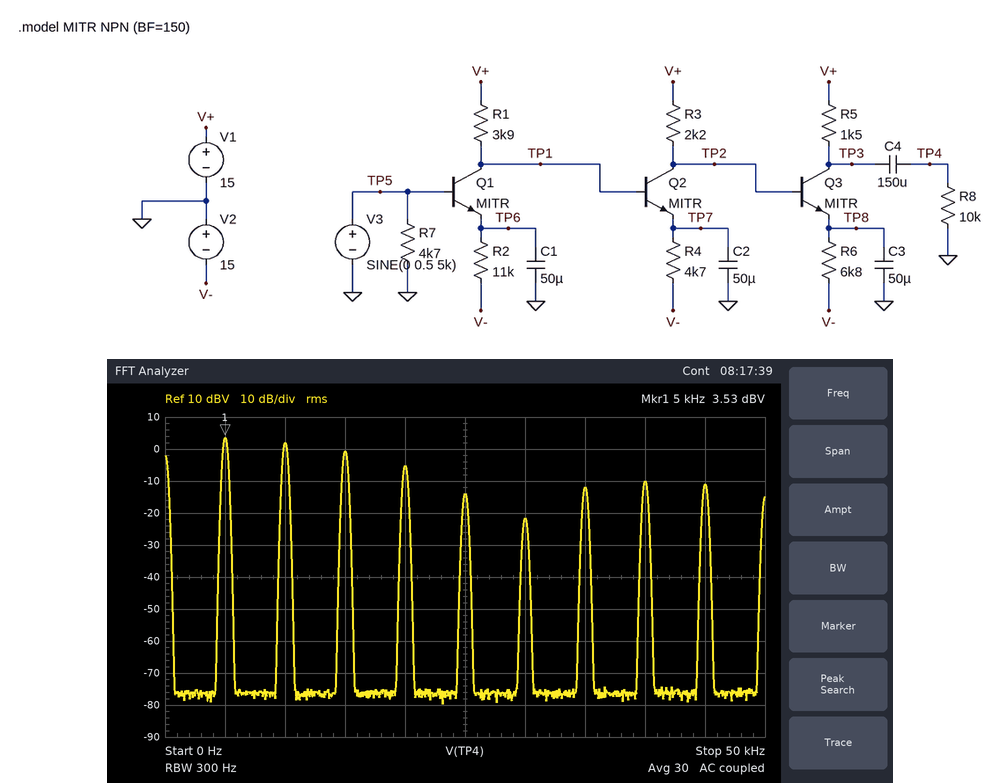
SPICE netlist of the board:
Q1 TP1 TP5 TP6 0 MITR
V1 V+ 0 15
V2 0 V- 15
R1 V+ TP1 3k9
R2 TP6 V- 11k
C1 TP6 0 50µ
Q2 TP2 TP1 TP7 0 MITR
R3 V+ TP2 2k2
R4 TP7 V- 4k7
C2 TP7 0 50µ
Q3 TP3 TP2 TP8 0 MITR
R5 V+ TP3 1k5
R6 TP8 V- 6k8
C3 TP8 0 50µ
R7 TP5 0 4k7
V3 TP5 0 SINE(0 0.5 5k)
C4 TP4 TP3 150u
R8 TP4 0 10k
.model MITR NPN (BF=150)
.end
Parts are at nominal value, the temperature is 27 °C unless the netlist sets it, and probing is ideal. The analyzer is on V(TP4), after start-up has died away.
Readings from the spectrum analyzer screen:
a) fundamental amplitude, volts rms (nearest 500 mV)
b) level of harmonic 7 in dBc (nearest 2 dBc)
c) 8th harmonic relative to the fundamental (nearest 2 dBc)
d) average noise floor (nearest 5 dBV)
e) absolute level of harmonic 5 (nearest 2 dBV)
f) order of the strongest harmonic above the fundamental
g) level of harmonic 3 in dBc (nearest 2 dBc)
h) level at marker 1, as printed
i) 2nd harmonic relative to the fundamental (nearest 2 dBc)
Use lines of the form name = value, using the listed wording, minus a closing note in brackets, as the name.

fundamental amplitude, volts rms = 1.5 V
level of harmonic 7 in dBc = -16 dBc
8th harmonic relative to the fundamental = -14 dBc
average noise floor = -75 dBV
absolute level of harmonic 5 = -14 dBV
order of the strongest harmonic above the fundamental = 2
level of harmonic 3 in dBc = -4 dBc
level at marker 1, as printed = 3.53 dBV
2nd harmonic relative to the fundamental = -2 dBc
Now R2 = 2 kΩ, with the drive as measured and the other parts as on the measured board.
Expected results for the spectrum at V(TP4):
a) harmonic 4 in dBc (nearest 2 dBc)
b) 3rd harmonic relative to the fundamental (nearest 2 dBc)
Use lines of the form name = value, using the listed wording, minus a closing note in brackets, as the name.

harmonic 4 in dBc = -12 dBc
3rd harmonic relative to the fundamental = -6 dBc
